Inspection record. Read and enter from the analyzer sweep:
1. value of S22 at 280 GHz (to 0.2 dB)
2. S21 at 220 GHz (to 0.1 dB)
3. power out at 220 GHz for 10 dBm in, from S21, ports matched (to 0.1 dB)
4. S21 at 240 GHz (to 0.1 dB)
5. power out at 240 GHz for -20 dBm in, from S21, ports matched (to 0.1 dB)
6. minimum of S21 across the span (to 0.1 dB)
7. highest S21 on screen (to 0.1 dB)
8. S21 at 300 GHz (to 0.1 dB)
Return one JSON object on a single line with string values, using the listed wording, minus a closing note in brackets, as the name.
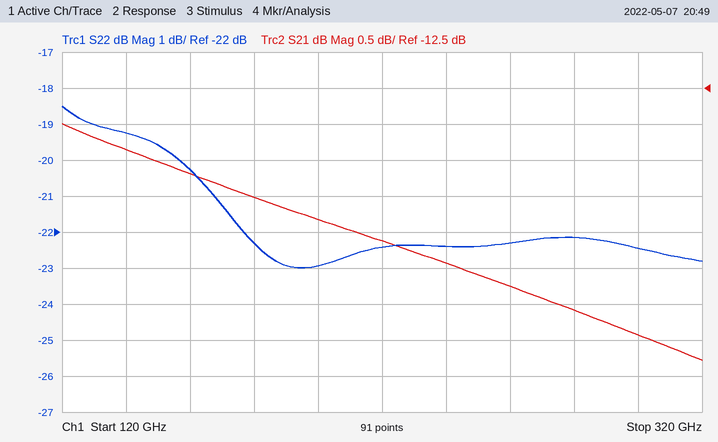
{"value of S22 at 280 GHz": "-22.2 dB", "S21 at 220 GHz": "-14.6 dB", "power out at 220 GHz for 10 dBm in, from S21, ports matched": "-4.6 dBm", "S21 at 240 GHz": "-14.9 dB", "power out at 240 GHz for -20 dBm in, from S21, ports matched": "-34.9 dBm", "minimum of S21 across the span": "-16.3 dB", "highest S21 on screen": "-13.0 dB", "S21 at 300 GHz": "-15.9 dB"}
